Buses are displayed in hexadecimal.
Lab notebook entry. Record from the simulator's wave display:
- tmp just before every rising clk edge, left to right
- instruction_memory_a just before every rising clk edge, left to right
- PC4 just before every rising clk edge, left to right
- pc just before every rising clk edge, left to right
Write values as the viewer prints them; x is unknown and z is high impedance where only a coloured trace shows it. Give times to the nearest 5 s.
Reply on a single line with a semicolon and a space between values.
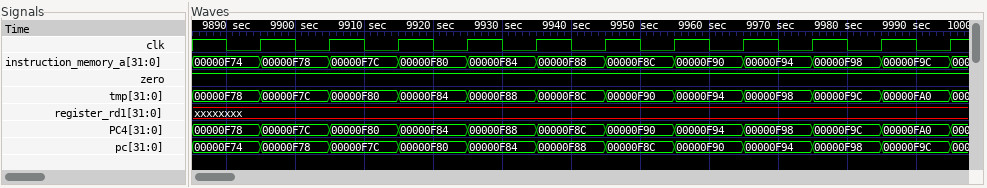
00000F78, 00000F7C, 00000F80, 00000F84, 00000F88, 00000F8C, 00000F90, 00000F94, 00000F98, 00000F9C, 00000FA0; 00000F74, 00000F78, 00000F7C, 00000F80, 00000F84, 00000F88, 00000F8C, 00000F90, 00000F94, 00000F98, 00000F9C; 00000F78, 00000F7C, 00000F80, 00000F84, 00000F88, 00000F8C, 00000F90, 00000F94, 00000F98, 00000F9C, 00000FA0; 00000F74, 00000F78, 00000F7C, 00000F80, 00000F84, 00000F88, 00000F8C, 00000F90, 00000F94, 00000F98, 00000F9C
